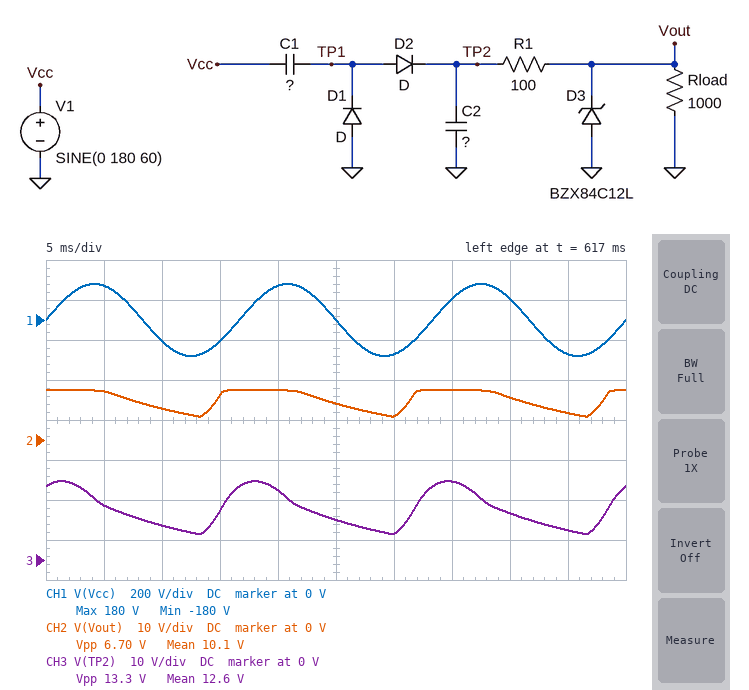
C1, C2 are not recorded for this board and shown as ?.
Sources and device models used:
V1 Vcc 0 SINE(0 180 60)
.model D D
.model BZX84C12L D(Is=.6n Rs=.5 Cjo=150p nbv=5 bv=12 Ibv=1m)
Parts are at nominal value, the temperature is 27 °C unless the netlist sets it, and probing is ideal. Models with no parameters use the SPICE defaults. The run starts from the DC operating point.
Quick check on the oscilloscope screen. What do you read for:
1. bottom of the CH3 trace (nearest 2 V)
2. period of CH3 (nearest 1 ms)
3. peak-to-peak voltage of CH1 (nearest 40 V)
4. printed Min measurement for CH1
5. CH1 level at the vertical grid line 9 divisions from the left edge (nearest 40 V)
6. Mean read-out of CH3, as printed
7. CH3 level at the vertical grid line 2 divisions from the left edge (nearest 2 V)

6 V
17 ms
360 V
-180 V
-160 V
12.6 V
8 V
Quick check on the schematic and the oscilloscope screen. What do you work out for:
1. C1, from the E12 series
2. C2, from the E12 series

1.2 µF
10 µF
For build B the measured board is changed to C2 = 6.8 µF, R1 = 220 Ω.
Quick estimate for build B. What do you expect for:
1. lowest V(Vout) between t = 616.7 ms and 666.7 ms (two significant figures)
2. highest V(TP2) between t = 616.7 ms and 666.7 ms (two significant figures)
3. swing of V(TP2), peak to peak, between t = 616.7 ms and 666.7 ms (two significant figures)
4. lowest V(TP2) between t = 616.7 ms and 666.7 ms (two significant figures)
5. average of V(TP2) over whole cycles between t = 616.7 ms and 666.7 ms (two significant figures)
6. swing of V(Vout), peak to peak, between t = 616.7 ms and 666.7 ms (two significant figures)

5.0 V
27 V
21 V
6.1 V
15 V
7.5 V
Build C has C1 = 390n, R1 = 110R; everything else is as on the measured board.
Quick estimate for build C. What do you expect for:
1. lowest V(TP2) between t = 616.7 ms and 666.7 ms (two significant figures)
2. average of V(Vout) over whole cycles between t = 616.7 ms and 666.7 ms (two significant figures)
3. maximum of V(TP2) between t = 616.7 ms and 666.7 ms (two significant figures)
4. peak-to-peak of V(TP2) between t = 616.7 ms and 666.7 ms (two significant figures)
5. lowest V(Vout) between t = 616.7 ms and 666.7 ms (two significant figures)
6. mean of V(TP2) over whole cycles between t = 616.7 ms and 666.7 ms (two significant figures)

5.4 V
8.1 V
13 V
7.4 V
4.9 V
9.0 V
